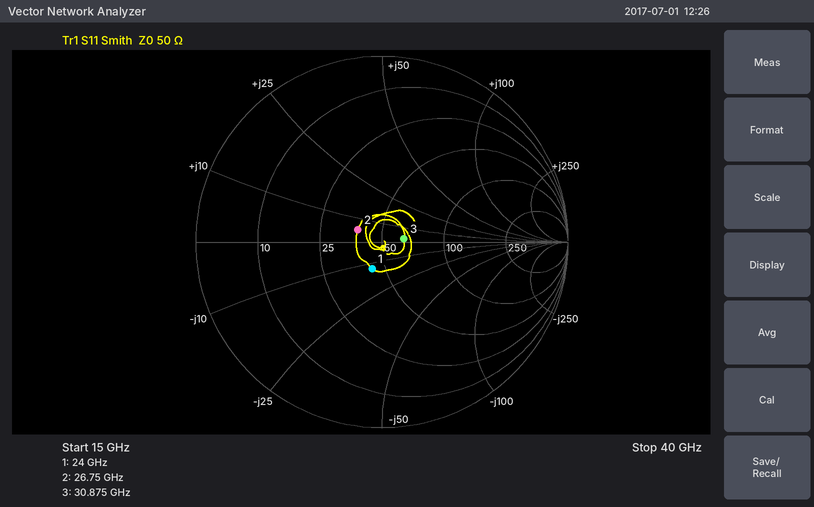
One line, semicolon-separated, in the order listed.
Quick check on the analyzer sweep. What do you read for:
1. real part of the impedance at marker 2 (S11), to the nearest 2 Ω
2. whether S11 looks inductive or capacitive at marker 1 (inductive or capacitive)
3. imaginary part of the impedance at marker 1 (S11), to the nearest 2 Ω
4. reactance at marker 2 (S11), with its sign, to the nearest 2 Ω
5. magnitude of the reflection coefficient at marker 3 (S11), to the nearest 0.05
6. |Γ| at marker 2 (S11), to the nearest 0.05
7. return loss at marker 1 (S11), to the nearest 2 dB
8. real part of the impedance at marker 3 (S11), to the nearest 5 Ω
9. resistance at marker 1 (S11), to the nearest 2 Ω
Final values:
38 Ω; capacitive; -12 Ω; +6 Ω; 0.10; 0.15; 16 dB; 65 Ω; 44 Ω
